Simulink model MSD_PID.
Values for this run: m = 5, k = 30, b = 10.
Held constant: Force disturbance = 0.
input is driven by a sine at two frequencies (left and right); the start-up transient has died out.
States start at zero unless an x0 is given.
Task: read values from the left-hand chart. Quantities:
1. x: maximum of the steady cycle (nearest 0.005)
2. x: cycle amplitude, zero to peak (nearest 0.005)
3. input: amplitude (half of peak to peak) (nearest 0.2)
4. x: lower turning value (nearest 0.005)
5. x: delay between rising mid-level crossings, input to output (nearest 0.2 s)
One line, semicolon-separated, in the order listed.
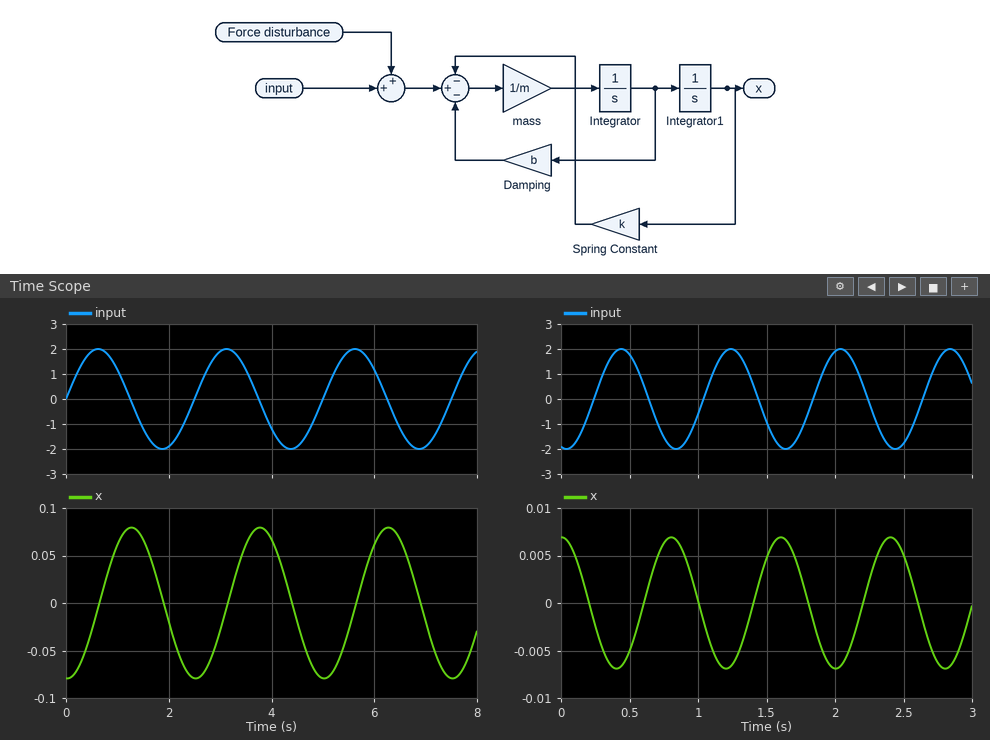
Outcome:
0.080; 0.080; 2.0; -0.080; 0.6 s
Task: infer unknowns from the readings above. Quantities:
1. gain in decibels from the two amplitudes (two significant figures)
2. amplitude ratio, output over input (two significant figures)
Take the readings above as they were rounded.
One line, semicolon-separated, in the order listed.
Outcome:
-28 dB; 0.040
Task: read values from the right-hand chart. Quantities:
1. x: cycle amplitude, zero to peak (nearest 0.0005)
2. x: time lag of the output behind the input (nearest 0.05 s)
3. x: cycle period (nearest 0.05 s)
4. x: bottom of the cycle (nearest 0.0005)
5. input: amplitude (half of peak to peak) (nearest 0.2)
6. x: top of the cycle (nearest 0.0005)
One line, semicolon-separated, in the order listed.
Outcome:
0.0070; 0.35 s; 0.80 s; -0.0070; 2.0; 0.0070
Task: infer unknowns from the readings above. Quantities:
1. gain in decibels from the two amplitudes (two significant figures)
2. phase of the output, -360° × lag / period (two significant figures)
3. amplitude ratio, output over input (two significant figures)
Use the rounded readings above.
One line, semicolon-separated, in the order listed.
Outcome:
-49 dB; -160°; 0.0035
